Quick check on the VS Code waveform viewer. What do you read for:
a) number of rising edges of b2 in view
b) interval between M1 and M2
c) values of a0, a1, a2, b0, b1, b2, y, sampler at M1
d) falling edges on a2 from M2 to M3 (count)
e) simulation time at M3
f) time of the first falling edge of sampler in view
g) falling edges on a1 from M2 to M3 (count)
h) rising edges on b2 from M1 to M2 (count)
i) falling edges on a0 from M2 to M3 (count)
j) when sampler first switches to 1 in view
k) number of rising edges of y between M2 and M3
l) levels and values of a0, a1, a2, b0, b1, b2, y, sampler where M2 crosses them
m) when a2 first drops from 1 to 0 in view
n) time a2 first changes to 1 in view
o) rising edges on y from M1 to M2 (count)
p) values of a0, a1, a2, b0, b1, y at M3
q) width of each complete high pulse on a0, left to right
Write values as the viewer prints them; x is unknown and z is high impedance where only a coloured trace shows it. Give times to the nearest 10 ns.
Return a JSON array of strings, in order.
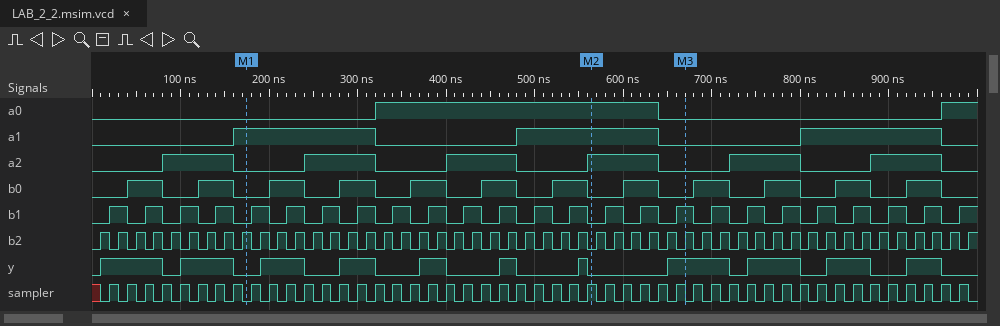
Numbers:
["50", "390 ns", "a0=0, a1=1, a2=0, b0=0, b1=0, b2=1, y=0, sampler=0", "1", "670 ns", "30 ns", "1", "19", "1", "20 ns", "1", "a0=1, a1=1, a2=1, b0=0, b1=0, b2=0, y=0, sampler=1", "160 ns", "80 ns", "5", "a0=0, a1=0, a2=0, b0=0, b1=1, y=1", "320 ns"]
